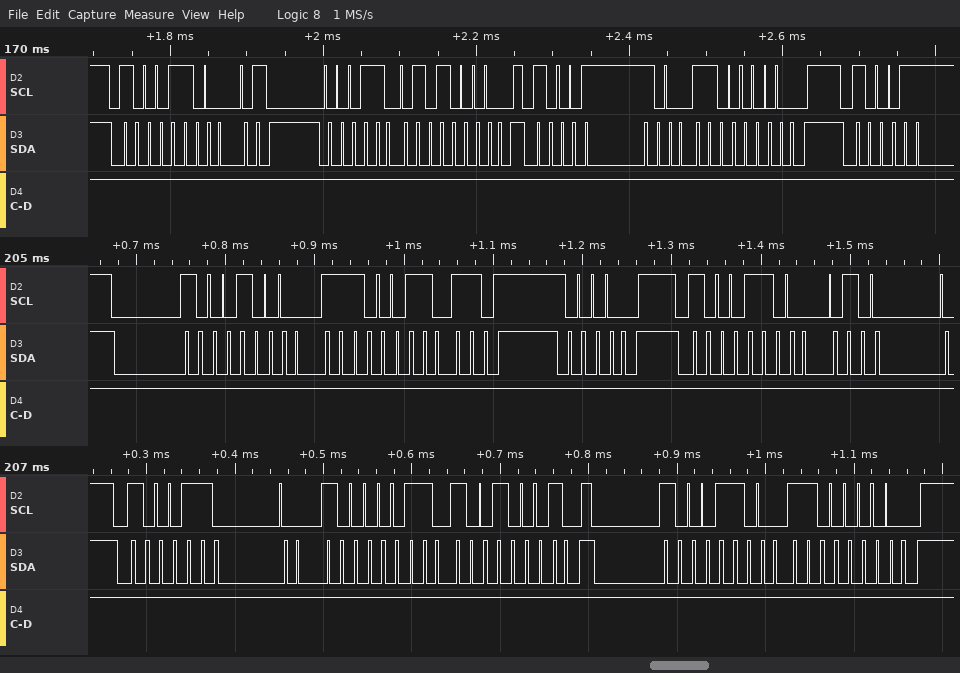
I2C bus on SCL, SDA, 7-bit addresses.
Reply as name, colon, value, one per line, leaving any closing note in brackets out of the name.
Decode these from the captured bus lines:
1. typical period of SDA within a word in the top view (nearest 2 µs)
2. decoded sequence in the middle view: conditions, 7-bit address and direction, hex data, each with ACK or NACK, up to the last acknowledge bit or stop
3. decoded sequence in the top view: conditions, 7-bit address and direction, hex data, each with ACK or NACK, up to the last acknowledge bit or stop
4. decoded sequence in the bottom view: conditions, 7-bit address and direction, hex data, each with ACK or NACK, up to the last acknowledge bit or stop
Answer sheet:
typical period of SDA within a word in the top view: 16 µs
decoded sequence in the middle view: conditions, 7-bit address and direction, hex data, each with ACK or NACK, up to the last acknowledge bit or stop: start, address 44 write ACK, E3 ACK, D0 ACK, stop, start, address 46 write ACK
decoded sequence in the top view: conditions, 7-bit address and direction, hex data, each with ACK or NACK, up to the last acknowledge bit or stop: start, address 46 write ACK, 43 ACK, 50 ACK, stop, start, address 46 write ACK, C0 ACK, stop
decoded sequence in the bottom view: conditions, 7-bit address and direction, hex data, each with ACK or NACK, up to the last acknowledge bit or stop: start, address 46 write ACK, 83 ACK, 91 ACK, stop, start, address 46 write ACK, C0 ACK, stop
